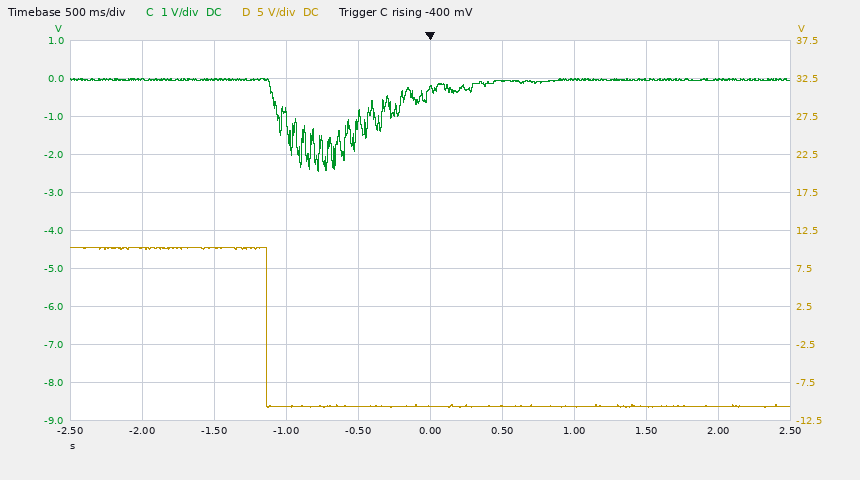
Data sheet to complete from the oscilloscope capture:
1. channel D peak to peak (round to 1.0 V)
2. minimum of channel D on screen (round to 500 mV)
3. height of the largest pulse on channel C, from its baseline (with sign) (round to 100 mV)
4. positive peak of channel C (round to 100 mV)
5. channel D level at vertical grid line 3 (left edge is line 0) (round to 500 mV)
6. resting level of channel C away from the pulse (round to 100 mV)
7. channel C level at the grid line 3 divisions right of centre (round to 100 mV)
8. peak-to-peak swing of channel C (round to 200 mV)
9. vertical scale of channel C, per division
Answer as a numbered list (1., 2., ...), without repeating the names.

1. 21.0 V
2. -11.0 V
3. -2.4 V
4. 0.0 V
5. -10.5 V
6. 0.0 V
7. 0.0 V
8. 2.4 V
9. 1 V
